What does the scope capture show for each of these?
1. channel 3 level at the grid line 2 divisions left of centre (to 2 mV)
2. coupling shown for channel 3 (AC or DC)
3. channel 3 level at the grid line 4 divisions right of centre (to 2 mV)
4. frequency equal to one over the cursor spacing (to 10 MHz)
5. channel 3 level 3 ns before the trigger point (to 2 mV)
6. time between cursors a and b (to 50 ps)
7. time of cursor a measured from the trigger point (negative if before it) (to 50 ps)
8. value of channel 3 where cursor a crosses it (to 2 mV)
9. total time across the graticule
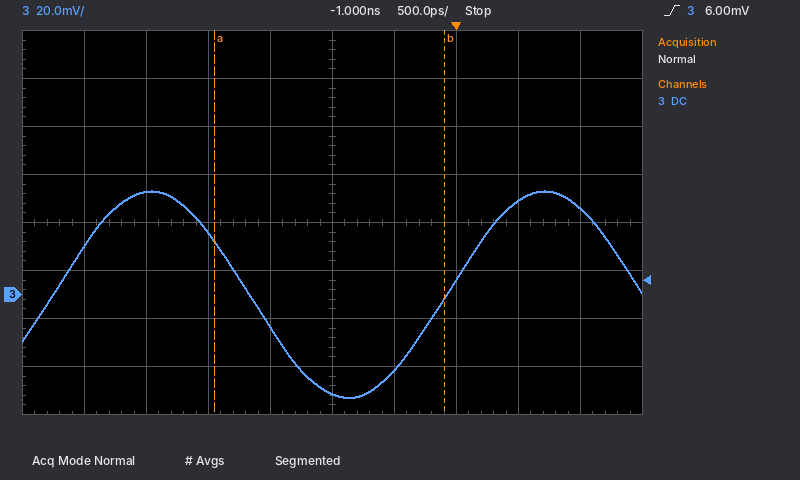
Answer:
26 mV
DC
36 mV
540 MHz
20 mV
1.85 ns
-1.95 ns
22 mV
5 ns
